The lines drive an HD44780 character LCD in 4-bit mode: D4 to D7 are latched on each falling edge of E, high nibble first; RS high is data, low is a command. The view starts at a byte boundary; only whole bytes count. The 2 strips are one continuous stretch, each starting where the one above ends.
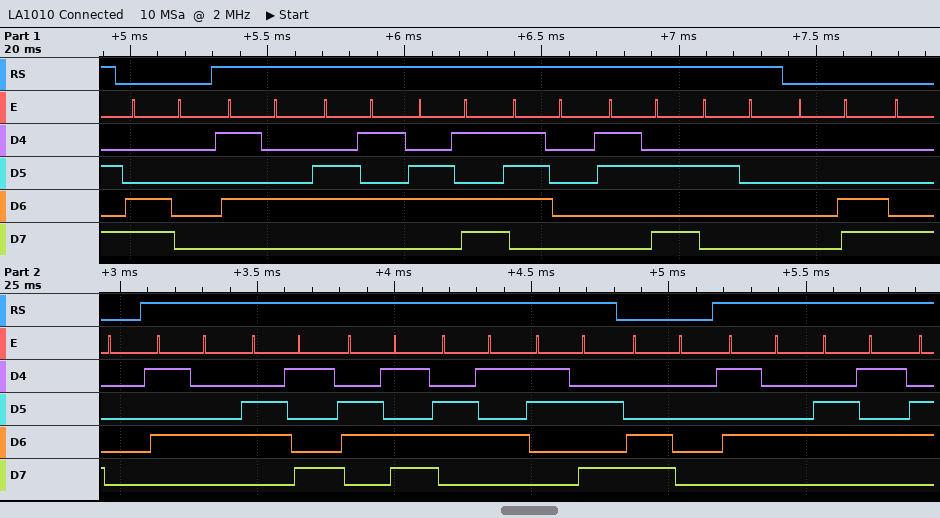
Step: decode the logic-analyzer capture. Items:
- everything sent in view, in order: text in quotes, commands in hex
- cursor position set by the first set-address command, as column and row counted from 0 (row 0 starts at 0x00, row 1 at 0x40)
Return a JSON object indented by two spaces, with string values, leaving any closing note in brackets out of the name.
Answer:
{
  "everything sent in view, in order: text in quotes, commands in hex": "0xC0 \"Temp: \" 0x0C 0x80 \"Time:\" 0xC0 \"Te\"",
  "cursor position set by the first set-address command, as column and row counted from 0": "column 0, row 1"
}
